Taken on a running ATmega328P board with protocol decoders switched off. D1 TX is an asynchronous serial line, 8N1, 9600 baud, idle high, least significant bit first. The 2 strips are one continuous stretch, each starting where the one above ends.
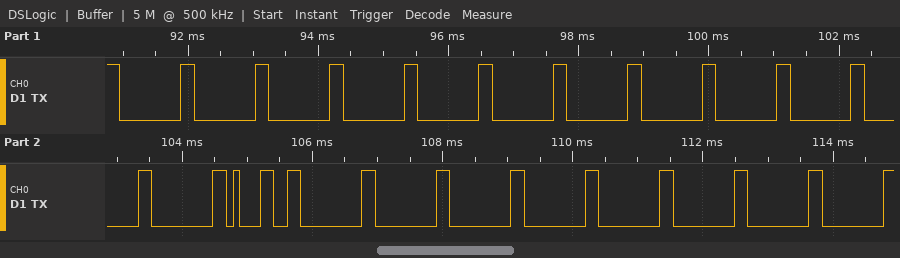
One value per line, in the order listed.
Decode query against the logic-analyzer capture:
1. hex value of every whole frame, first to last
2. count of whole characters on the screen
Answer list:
0x00 0x00 0x00 0x00 0x00 0x00 0x00 0x00 0x00 0x00 0x00 0x00 0x31 0x00 0x00 0x00 0x00 0x00 0x00 0x00 0x00
21
